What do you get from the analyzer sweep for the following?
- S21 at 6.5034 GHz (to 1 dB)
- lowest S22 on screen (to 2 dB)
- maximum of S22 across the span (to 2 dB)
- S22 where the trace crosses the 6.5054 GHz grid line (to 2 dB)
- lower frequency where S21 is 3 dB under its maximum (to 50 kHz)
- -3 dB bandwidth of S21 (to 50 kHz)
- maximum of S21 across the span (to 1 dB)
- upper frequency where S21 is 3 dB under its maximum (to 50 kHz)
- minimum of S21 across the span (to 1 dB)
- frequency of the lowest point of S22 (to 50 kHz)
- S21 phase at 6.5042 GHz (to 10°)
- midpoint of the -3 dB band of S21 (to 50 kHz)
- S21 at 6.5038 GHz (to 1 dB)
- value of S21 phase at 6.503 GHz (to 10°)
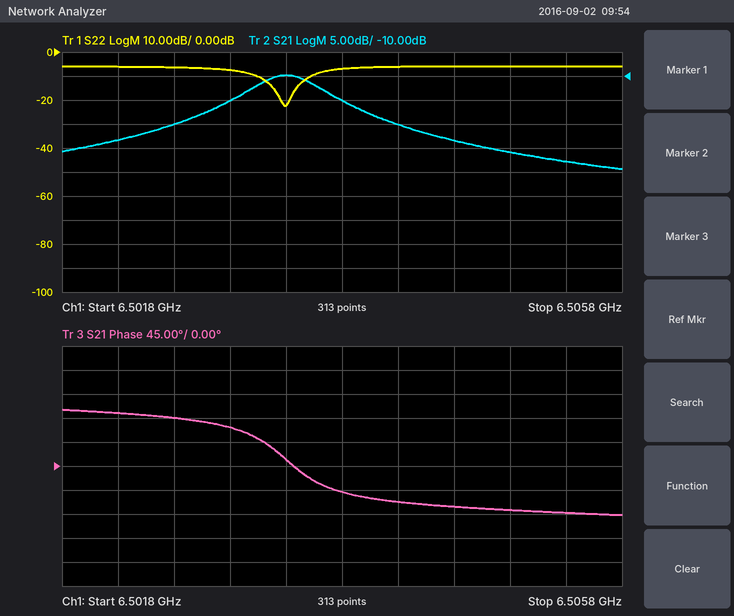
-10 dB
-22 dB
-6 dB
-6 dB
6.50315 GHz
500 kHz
-10 dB
6.50365 GHz
-29 dB
6.50340 GHz
-70°
6.50340 GHz
-15 dB
70°
